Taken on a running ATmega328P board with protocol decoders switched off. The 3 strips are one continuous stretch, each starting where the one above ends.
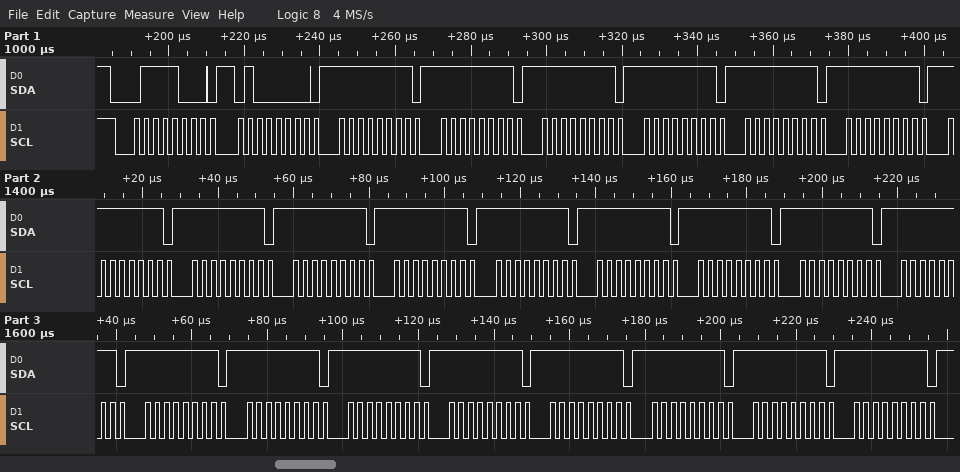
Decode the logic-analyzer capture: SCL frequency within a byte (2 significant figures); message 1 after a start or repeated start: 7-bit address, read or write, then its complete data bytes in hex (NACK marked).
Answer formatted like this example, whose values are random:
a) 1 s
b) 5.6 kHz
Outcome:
a) 400 kHz
b) 0x3C write: 40 FF FF FF FF FF FF FF FF FF FF FF FF FF FF FF FF FF FF FF FF FF FF FF
